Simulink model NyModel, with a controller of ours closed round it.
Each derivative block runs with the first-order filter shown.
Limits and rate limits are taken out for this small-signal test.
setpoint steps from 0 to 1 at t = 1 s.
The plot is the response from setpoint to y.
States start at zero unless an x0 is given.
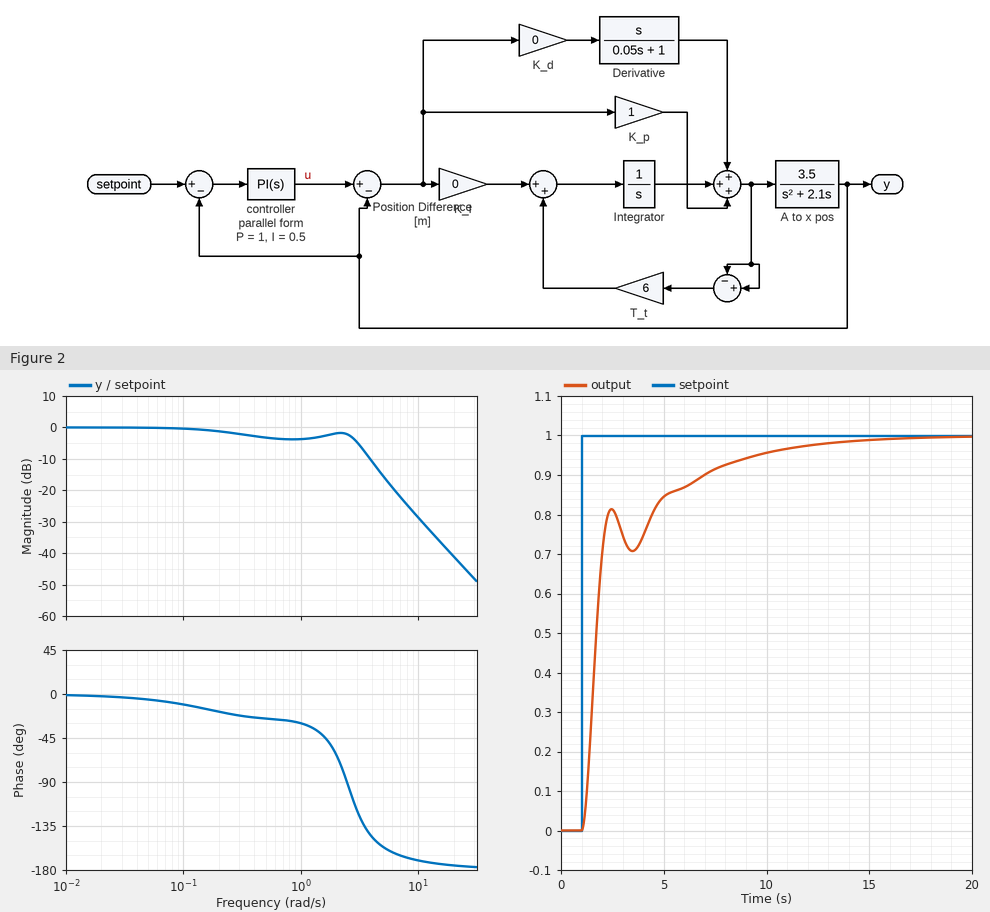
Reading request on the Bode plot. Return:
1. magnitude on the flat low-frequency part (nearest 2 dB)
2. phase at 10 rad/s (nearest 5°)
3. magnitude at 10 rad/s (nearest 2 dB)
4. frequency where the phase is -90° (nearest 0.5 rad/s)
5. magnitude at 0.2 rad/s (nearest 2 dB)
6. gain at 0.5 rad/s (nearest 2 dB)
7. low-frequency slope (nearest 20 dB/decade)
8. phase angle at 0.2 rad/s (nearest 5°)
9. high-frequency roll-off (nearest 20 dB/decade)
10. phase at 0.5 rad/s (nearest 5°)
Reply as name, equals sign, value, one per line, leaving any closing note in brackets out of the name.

magnitude on the flat low-frequency part = 0 dB
phase at 10 rad/s = -170°
magnitude at 10 rad/s = -28 dB
frequency where the phase is -90° = 2.5 rad/s
magnitude at 0.2 rad/s = -2 dB
gain at 0.5 rad/s = -4 dB
low-frequency slope = 0 dB/decade
phase angle at 0.2 rad/s = -20°
high-frequency roll-off = -40 dB/decade
phase at 0.5 rad/s = -25°
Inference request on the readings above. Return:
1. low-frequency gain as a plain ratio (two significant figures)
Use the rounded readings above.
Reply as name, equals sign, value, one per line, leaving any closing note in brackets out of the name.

low-frequency gain as a plain ratio = 1.0
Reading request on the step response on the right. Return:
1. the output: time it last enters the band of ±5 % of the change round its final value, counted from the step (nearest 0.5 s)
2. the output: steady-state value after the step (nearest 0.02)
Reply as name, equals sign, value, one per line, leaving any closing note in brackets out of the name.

the output: time it last enters the band of ±5 % of the change round its final value, counted from the step = 8.5 s
the output: steady-state value after the step = 1.00
